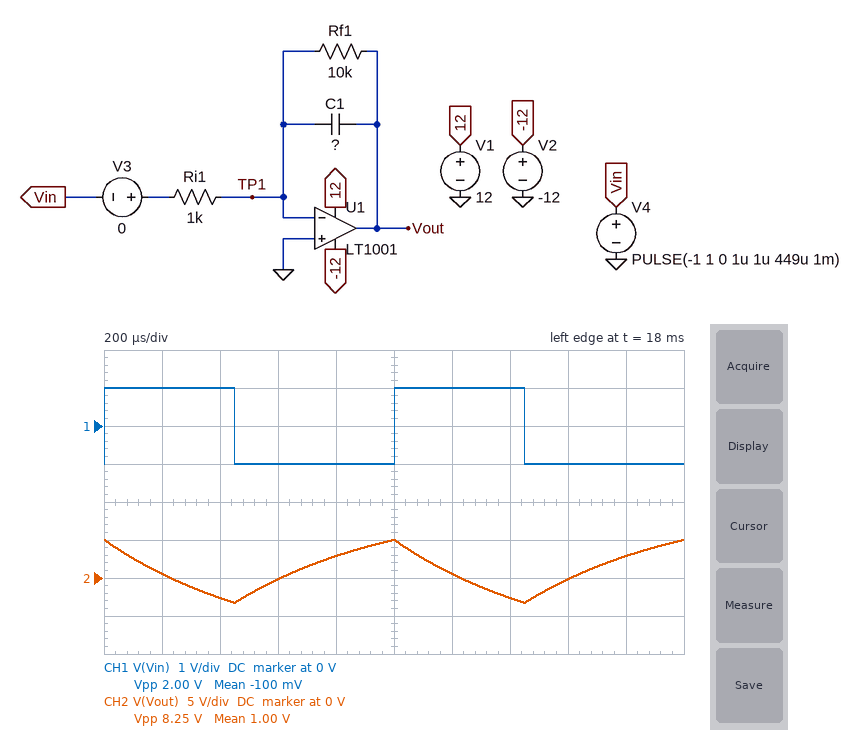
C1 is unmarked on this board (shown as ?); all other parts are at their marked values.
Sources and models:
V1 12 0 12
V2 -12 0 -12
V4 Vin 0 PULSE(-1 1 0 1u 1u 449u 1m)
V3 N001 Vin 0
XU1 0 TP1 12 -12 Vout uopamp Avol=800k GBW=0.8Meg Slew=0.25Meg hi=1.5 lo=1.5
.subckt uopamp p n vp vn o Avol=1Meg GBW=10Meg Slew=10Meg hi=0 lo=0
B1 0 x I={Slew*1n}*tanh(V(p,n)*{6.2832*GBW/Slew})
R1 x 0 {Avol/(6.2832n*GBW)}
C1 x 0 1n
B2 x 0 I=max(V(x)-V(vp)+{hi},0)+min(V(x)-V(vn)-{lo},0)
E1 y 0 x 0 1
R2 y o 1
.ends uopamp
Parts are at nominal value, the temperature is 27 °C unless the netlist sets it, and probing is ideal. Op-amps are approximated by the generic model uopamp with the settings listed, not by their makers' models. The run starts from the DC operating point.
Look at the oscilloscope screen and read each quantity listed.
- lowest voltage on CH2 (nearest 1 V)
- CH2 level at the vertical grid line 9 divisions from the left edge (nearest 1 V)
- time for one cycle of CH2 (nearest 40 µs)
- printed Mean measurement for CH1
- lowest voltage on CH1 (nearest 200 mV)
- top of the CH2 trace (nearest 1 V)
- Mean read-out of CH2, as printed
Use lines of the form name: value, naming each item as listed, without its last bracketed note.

lowest voltage on CH2: -3 V
CH2 level at the vertical grid line 9 divisions from the left edge: 3 V
time for one cycle of CH2: 1.00 ms
printed Mean measurement for CH1: -100 mV
lowest voltage on CH1: -1.0 V
top of the CH2 trace: 5 V
Mean read-out of CH2, as printed: 1.00 V
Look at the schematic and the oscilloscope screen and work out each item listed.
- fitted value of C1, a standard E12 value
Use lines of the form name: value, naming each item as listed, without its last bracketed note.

fitted value of C1, a standard E12 value: 56 nF
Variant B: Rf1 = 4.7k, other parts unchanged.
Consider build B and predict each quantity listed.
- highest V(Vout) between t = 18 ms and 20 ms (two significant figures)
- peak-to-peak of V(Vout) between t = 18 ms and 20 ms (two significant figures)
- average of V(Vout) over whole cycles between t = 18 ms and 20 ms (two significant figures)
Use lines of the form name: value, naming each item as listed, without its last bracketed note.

highest V(Vout) between t = 18 ms and 20 ms: 3.7 V
peak-to-peak of V(Vout) between t = 18 ms and 20 ms: 6.9 V
average of V(Vout) over whole cycles between t = 18 ms and 20 ms: 470 mV
